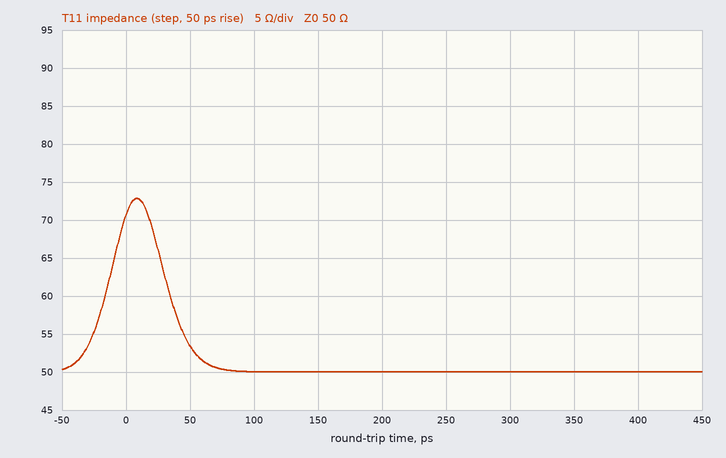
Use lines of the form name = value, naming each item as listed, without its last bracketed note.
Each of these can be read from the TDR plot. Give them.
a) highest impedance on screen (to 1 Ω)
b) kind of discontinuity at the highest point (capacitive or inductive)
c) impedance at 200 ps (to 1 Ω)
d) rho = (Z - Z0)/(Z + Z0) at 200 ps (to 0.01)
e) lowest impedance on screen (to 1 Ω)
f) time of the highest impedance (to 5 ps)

highest impedance on screen = 73 Ω
kind of discontinuity at the highest point = inductive
impedance at 200 ps = 50 Ω
rho = (Z - Z0)/(Z + Z0) at 200 ps = 0.00
lowest impedance on screen = 50 Ω
time of the highest impedance = 10 ps
